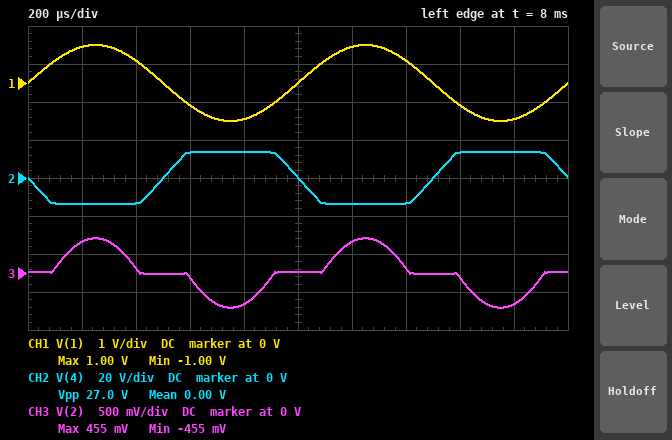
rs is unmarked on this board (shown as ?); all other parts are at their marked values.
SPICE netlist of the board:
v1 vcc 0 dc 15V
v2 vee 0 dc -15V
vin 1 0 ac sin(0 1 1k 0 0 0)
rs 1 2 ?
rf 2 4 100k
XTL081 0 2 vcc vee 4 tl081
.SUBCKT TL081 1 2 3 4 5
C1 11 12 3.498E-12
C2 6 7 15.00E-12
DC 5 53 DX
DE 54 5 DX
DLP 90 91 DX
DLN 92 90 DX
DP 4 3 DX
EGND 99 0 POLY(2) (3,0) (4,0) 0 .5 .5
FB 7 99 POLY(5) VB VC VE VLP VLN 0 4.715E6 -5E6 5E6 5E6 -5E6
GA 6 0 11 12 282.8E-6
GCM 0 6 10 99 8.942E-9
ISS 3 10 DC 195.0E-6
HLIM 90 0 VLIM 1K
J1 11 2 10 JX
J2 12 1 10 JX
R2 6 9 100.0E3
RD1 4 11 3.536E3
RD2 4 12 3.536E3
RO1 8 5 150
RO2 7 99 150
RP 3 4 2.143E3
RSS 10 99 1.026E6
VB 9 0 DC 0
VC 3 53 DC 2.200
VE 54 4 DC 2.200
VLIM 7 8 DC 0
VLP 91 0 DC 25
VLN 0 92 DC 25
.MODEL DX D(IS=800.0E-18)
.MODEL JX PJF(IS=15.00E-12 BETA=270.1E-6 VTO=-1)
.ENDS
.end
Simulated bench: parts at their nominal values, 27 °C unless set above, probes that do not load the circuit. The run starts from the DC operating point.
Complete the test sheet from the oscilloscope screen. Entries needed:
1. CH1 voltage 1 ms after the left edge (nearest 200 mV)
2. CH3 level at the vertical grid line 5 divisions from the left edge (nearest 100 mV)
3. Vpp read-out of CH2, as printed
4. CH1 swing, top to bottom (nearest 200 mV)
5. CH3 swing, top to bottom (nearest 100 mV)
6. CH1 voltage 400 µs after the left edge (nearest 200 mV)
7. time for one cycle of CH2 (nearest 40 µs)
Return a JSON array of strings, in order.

["0 V", "0 V", "27.0 V", "2.0 V", "900 mV", "600 mV", "1.00 ms"]
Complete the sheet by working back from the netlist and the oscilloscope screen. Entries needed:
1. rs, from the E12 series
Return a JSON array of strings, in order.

["3.9 kΩ"]
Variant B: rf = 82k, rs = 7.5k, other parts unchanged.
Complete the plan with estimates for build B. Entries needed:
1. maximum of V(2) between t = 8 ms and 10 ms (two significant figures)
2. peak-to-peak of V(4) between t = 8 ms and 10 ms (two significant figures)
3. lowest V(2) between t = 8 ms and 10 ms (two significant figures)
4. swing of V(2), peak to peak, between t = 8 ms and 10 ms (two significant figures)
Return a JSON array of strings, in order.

["3.2 mV", "22 V", "-3.2 mV", "6.4 mV"]
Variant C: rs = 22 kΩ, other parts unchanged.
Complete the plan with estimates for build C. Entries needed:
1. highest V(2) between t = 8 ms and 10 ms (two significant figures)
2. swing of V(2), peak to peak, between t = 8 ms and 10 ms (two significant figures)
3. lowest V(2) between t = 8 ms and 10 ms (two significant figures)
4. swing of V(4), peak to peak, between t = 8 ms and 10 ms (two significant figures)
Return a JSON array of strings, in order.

["1.3 mV", "2.6 mV", "-1.3 mV", "9.1 V"]
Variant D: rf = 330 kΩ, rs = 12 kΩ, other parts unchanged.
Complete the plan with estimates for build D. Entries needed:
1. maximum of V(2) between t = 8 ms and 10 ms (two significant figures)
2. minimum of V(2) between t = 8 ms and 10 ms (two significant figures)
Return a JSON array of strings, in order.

["490 mV", "-490 mV"]
